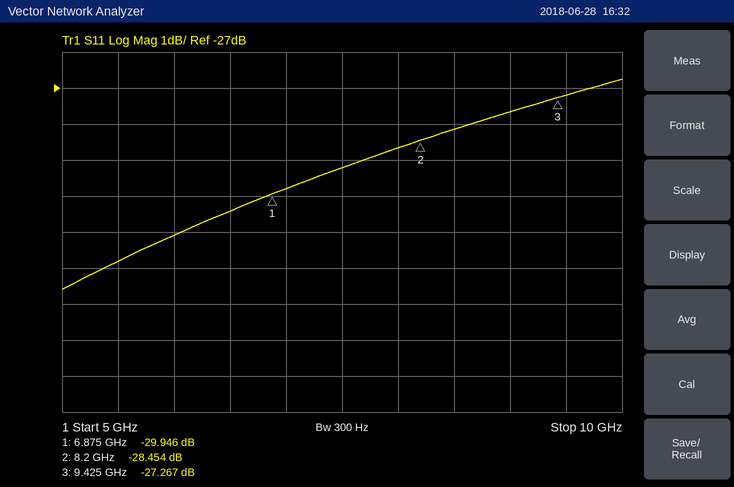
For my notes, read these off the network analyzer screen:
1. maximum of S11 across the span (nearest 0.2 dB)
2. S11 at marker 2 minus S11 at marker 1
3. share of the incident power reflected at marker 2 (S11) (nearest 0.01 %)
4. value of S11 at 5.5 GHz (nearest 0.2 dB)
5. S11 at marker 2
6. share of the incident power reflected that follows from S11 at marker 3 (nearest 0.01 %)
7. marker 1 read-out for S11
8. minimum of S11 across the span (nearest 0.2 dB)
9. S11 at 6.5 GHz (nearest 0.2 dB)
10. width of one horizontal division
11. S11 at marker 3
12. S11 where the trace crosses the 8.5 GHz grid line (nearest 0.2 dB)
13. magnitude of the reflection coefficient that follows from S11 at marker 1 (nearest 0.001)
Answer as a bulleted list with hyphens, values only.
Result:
- -26.8 dB
- 1.492 dB
- 0.14 %
- -31.8 dB
- -28.454 dB
- 0.19 %
- -29.946 dB
- -32.6 dB
- -30.4 dB
- 500 MHz
- -27.267 dB
- -28.2 dB
- 0.032
